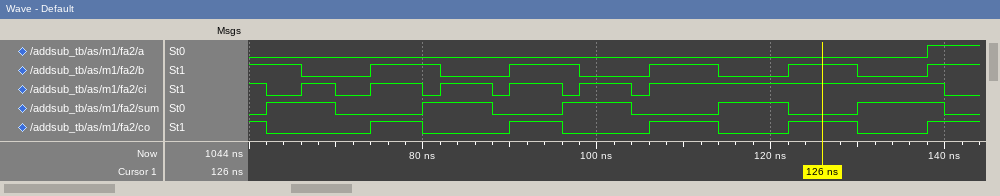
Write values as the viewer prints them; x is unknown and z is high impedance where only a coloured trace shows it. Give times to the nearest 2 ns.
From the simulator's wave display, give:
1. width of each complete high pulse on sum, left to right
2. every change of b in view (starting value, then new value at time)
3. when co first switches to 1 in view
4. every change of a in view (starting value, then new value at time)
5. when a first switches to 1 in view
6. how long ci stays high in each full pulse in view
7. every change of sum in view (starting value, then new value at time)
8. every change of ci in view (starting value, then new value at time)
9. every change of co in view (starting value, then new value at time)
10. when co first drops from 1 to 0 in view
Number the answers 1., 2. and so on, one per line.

1. 8 ns, 8 ns, 8 ns, 8 ns, 10 ns
2. 1, 0 at 66 ns, 1 at 74 ns, 0 at 82 ns, 1 at 90 ns, 0 at 98 ns, 1 at 106 ns, 0 at 114 ns, 1 at 122 ns, 0 at 130 ns, 1 at 138 ns
3. 74 ns
4. 0, 1 at 138 ns
5. 138 ns
6. 4 ns, 6 ns, 6 ns, 6 ns, 6 ns, 34 ns
7. 0, 1 at 62 ns, 0 at 70 ns, 1 at 80 ns, 0 at 88 ns, 1 at 96 ns, 0 at 104 ns, 1 at 114 ns, 0 at 122 ns, 1 at 130 ns, 0 at 140 ns
8. 1, 0 at 62 ns, 1 at 66 ns, 0 at 70 ns, 1 at 74 ns, 0 at 80 ns, 1 at 82 ns, 0 at 88 ns, 1 at 90 ns, 0 at 96 ns, 1 at 98 ns, 0 at 104 ns, 1 at 106 ns, 0 at 140 ns
9. 1, 0 at 62 ns, 1 at 74 ns, 0 at 80 ns, 1 at 90 ns, 0 at 96 ns, 1 at 106 ns, 0 at 114 ns, 1 at 122 ns, 0 at 130 ns, 1 at 138 ns
10. 62 ns
